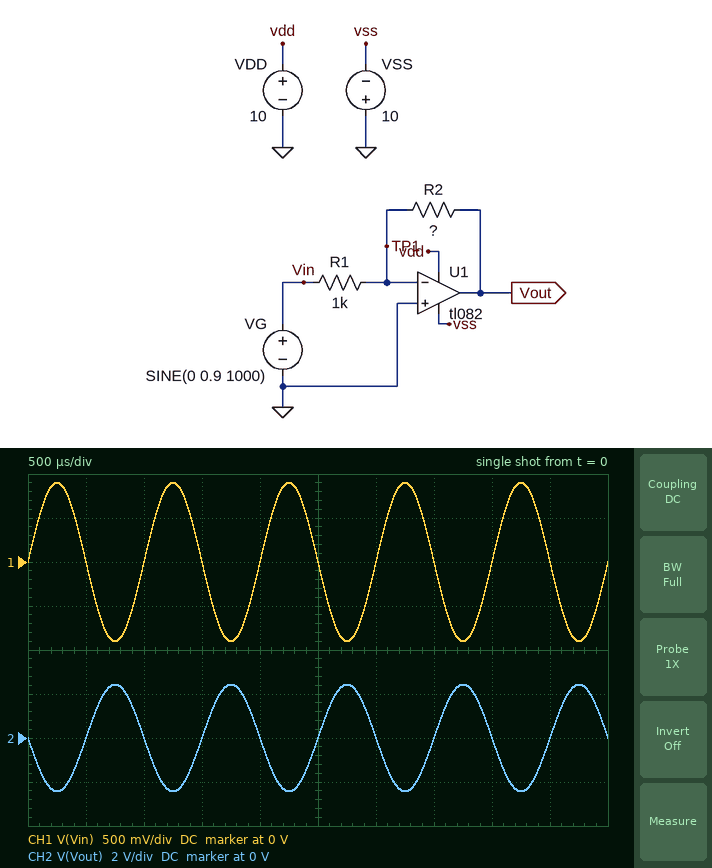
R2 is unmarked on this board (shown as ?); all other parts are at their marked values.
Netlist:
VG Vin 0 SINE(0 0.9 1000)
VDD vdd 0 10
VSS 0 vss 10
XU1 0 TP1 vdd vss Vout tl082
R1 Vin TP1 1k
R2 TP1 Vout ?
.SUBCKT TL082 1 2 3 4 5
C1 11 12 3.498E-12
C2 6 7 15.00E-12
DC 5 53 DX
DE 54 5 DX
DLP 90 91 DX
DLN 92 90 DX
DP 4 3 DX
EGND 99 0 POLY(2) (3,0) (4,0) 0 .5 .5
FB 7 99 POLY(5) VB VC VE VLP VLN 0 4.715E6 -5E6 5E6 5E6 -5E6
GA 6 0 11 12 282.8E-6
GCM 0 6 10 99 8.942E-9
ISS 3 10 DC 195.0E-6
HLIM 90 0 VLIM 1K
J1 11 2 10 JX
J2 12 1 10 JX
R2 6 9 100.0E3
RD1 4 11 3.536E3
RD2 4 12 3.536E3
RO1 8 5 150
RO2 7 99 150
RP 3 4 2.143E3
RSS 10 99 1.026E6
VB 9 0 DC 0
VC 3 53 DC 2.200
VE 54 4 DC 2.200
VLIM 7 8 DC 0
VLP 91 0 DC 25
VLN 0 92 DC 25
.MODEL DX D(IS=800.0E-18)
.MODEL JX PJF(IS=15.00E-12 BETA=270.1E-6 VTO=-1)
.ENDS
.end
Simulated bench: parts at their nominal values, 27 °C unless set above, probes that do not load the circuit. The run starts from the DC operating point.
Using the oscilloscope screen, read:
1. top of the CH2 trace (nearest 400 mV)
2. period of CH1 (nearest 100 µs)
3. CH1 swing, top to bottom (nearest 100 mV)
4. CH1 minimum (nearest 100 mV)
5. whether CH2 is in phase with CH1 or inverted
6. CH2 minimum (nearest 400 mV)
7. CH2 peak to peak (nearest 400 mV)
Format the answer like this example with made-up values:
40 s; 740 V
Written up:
2.4 V; 1.0 ms; 1.8 V; -900 mV; inverted; -2.4 V; 4.8 V
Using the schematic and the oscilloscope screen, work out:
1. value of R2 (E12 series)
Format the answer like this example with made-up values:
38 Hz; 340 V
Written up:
2.7 kΩ
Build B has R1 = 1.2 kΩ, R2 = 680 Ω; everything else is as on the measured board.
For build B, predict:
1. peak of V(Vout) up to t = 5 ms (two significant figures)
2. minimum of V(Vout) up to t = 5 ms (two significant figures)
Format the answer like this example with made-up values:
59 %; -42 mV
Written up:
510 mV; -510 mV
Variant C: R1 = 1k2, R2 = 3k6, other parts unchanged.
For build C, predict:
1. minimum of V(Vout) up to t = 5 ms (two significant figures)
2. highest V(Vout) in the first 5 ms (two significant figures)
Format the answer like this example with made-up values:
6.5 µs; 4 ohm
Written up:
-2.7 V; 2.7 V
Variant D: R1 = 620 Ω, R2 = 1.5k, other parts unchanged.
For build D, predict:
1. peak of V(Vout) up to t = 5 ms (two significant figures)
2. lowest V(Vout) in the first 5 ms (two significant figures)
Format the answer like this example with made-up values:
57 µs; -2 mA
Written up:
2.2 V; -2.2 V
